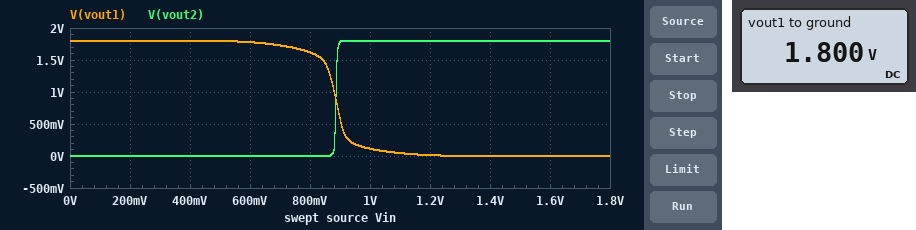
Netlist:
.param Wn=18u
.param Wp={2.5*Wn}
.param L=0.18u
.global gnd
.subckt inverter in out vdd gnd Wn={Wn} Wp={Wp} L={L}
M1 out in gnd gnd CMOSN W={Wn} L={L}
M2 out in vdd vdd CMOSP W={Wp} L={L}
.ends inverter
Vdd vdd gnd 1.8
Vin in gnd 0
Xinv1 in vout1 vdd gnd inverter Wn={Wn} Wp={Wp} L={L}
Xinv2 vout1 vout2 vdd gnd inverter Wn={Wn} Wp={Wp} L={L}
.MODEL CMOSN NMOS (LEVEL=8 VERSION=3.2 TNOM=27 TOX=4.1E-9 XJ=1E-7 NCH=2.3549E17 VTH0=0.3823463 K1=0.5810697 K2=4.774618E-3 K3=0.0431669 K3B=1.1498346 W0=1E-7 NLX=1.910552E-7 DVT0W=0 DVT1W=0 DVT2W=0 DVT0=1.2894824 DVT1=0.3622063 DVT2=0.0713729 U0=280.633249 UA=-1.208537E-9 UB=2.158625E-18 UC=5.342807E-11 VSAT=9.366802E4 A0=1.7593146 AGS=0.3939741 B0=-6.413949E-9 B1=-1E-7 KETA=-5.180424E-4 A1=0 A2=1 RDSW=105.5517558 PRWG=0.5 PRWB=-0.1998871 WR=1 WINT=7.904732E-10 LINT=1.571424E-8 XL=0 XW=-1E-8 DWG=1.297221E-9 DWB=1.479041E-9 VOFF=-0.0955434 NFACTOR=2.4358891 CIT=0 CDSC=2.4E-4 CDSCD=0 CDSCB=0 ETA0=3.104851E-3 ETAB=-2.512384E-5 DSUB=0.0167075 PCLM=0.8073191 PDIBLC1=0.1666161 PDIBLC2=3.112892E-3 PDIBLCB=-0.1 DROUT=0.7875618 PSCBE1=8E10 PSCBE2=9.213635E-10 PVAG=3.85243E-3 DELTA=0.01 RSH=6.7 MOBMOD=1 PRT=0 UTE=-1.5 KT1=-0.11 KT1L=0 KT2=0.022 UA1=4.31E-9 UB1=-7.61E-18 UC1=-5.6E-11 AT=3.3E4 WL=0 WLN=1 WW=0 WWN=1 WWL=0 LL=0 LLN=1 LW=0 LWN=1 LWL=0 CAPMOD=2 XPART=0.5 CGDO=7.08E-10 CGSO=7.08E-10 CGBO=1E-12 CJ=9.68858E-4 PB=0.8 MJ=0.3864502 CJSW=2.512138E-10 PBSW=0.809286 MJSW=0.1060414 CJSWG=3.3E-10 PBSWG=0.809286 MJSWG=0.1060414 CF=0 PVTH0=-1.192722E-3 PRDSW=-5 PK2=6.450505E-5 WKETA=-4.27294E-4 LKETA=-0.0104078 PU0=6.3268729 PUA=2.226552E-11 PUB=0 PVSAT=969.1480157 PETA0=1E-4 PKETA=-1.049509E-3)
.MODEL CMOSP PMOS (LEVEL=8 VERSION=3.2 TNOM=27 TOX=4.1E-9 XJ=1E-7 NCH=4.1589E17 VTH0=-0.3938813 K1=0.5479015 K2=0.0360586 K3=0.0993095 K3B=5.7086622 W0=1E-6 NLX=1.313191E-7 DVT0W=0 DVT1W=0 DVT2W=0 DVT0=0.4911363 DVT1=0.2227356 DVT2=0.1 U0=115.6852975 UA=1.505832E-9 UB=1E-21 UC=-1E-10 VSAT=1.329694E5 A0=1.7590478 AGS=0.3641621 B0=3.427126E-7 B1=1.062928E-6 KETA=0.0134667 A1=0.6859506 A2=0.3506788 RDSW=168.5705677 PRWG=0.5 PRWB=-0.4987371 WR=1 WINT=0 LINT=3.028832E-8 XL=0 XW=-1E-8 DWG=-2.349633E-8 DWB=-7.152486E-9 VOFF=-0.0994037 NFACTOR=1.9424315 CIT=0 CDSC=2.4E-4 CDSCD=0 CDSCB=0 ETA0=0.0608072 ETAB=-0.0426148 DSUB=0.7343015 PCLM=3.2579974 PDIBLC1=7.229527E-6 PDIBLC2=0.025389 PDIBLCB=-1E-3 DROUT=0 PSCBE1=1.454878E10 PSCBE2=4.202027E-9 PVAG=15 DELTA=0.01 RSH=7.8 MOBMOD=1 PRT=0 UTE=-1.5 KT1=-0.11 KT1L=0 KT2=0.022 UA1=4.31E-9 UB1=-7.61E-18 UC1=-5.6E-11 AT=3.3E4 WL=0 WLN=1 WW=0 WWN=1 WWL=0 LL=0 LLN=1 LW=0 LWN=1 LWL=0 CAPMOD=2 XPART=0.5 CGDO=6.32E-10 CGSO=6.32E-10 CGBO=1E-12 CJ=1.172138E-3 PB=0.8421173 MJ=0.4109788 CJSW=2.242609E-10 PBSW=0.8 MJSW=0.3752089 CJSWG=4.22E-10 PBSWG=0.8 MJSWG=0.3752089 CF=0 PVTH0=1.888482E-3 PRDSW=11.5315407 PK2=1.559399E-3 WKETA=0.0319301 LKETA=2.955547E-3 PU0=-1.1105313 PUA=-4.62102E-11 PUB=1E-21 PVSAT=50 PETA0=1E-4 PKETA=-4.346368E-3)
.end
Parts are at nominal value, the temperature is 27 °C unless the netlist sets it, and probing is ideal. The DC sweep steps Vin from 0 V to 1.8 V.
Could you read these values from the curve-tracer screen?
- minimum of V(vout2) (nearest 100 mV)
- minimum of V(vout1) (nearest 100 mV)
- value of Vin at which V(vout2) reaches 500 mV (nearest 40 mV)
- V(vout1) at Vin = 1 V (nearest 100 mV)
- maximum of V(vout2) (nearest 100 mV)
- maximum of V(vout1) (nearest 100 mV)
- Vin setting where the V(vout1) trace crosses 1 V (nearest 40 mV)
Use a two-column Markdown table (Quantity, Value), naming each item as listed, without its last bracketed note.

| Quantity | Value |
|---|---|
| minimum of V(vout2) | 0 V |
| minimum of V(vout1) | 0 V |
| value of Vin at which V(vout2) reaches 500 mV | 880 mV |
| V(vout1) at Vin = 1 V | 100 mV |
| maximum of V(vout2) | 1.8 V |
| maximum of V(vout1) | 1.8 V |
| Vin setting where the V(vout1) trace crosses 1 V | 880 mV |
